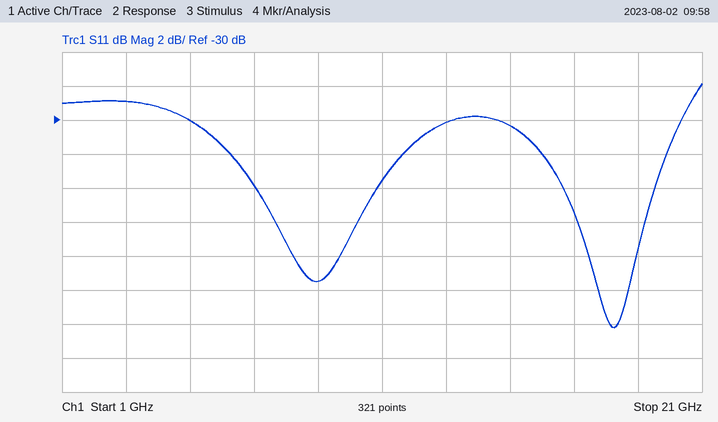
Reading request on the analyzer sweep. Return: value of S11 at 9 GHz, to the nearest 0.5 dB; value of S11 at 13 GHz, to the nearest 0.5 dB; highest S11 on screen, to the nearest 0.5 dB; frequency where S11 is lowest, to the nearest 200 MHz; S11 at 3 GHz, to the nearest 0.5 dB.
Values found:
-39.5 dB
-30.0 dB
-28.0 dB
18.2 GHz
-29.0 dB
